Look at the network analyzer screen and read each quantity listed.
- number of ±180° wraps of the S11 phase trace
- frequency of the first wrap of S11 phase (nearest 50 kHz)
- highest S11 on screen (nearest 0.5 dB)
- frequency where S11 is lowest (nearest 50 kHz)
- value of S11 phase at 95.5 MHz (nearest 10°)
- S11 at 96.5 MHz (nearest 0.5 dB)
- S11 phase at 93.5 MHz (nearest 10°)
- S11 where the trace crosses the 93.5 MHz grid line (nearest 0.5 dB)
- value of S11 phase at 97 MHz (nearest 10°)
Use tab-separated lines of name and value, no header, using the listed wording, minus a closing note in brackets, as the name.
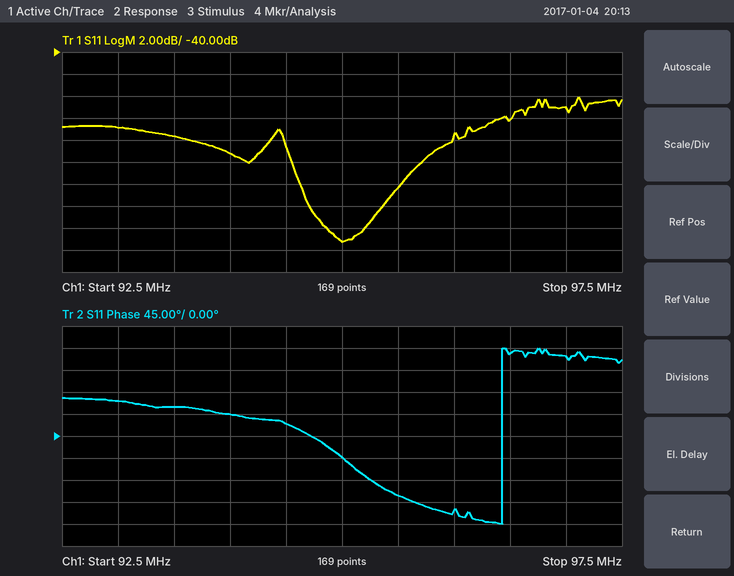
number of ±180° wraps of the S11 phase trace	1
frequency of the first wrap of S11 phase	96.45 MHz
highest S11 on screen	-44.0 dB
frequency where S11 is lowest	95.00 MHz
value of S11 phase at 95.5 MHz	-120°
S11 at 96.5 MHz	-46.0 dB
S11 phase at 93.5 MHz	60°
S11 where the trace crosses the 93.5 MHz grid line	-47.5 dB
value of S11 phase at 97 MHz	160°
